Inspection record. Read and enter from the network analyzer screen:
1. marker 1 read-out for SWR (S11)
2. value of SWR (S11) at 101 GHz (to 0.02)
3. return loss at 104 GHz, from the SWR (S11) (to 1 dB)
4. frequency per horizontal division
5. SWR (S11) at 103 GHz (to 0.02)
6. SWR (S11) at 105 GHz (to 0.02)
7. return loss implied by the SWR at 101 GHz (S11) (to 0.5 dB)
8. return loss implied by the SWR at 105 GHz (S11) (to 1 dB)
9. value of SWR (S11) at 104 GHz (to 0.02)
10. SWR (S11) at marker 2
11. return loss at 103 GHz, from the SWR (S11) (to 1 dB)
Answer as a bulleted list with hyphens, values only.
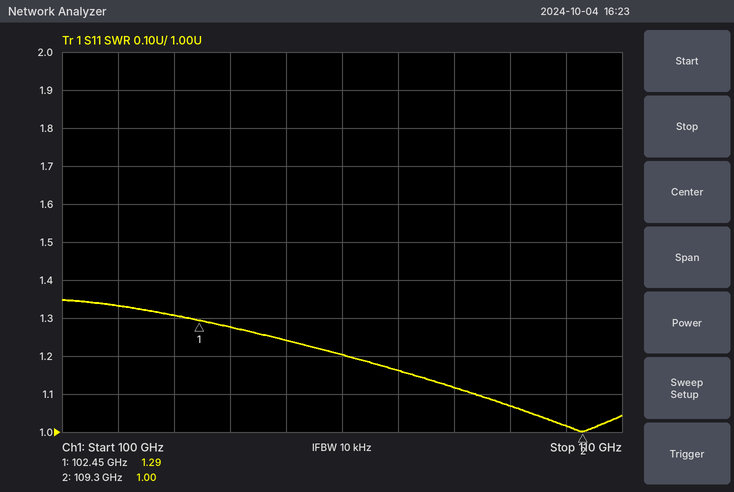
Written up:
- 1.29
- 1.34
- 19 dB
- 1 GHz
- 1.28
- 1.20
- 17.0 dB
- 21 dB
- 1.24
- 1.00
- 18 dB
